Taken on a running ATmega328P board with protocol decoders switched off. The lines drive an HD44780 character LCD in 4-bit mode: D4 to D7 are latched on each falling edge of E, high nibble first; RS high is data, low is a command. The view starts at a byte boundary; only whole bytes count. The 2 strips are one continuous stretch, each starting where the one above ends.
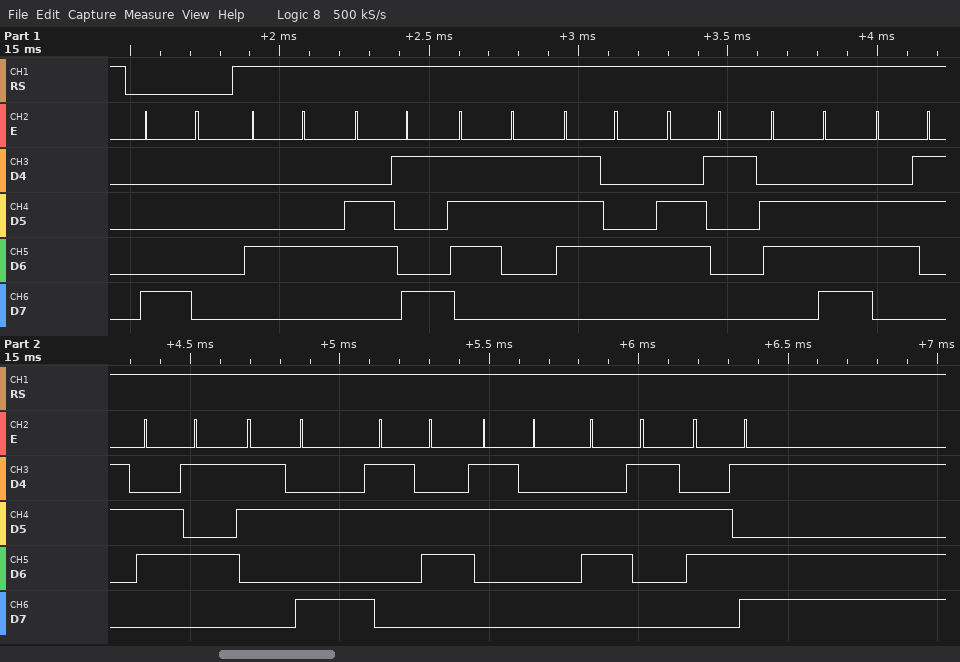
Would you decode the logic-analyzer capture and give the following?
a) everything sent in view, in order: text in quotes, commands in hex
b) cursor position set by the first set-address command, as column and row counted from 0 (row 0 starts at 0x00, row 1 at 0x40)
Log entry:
0x80 "Distance:62cm"
column 0, row 0
